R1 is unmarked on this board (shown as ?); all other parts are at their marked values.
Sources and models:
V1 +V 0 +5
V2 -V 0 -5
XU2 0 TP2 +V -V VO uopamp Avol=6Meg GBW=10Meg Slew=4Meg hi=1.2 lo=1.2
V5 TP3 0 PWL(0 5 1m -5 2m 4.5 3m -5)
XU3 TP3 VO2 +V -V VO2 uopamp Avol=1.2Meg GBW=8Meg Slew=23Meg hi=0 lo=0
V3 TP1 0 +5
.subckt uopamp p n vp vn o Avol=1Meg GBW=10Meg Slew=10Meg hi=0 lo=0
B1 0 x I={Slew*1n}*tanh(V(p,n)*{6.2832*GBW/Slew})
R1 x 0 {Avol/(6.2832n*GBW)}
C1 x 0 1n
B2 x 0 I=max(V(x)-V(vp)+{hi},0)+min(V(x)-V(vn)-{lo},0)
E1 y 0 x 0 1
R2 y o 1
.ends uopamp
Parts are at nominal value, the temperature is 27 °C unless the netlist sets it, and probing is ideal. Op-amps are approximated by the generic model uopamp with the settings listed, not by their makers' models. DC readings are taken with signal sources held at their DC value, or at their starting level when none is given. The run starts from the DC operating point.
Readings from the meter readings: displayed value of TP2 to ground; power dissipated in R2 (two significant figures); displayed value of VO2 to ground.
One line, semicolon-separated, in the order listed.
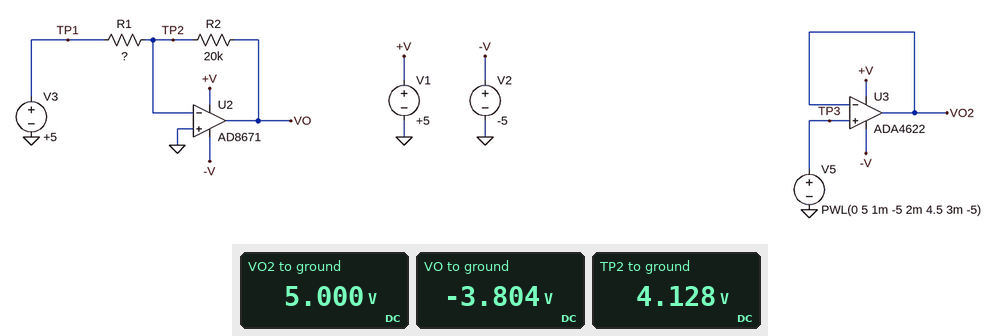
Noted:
4.128 V; 3.1 mW; 5.000 V
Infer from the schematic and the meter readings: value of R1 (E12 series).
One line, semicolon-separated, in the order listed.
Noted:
2.2 kΩ
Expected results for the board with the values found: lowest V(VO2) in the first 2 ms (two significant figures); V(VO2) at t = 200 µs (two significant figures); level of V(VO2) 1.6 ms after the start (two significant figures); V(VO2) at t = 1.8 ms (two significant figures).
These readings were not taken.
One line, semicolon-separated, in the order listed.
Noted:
-5.0 V; 3.0 V; 700 mV; 2.6 V
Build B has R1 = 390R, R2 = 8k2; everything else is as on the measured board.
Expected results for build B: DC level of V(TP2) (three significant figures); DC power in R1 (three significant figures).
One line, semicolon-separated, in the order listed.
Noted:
4.60 V; 410 µW
